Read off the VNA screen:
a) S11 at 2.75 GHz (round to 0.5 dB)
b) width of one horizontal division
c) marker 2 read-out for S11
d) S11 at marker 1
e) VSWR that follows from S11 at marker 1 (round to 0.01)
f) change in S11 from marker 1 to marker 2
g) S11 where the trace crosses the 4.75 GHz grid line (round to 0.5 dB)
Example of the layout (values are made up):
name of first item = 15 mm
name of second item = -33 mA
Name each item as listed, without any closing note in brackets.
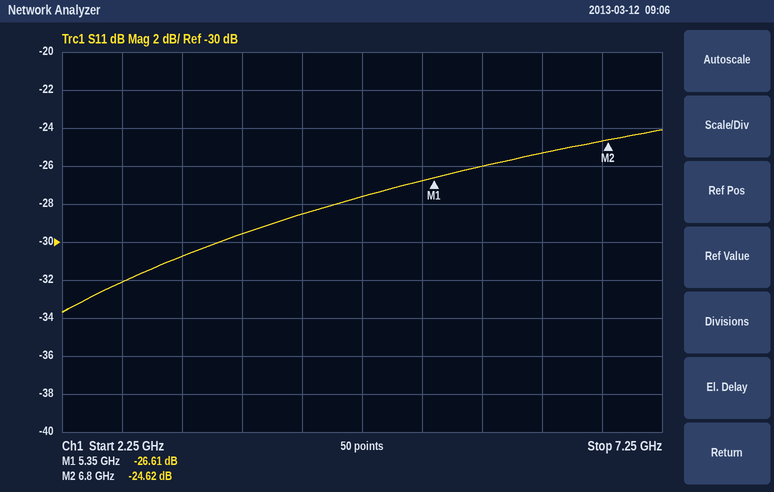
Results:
S11 at 2.75 GHz = -32.0 dB
width of one horizontal division = 500 MHz
marker 2 read-out for S11 = -24.62 dB
S11 at marker 1 = -26.61 dB
VSWR that follows from S11 at marker 1 = 1.10
change in S11 from marker 1 to marker 2 = 1.99 dB
S11 where the trace crosses the 4.75 GHz grid line = -27.5 dB
